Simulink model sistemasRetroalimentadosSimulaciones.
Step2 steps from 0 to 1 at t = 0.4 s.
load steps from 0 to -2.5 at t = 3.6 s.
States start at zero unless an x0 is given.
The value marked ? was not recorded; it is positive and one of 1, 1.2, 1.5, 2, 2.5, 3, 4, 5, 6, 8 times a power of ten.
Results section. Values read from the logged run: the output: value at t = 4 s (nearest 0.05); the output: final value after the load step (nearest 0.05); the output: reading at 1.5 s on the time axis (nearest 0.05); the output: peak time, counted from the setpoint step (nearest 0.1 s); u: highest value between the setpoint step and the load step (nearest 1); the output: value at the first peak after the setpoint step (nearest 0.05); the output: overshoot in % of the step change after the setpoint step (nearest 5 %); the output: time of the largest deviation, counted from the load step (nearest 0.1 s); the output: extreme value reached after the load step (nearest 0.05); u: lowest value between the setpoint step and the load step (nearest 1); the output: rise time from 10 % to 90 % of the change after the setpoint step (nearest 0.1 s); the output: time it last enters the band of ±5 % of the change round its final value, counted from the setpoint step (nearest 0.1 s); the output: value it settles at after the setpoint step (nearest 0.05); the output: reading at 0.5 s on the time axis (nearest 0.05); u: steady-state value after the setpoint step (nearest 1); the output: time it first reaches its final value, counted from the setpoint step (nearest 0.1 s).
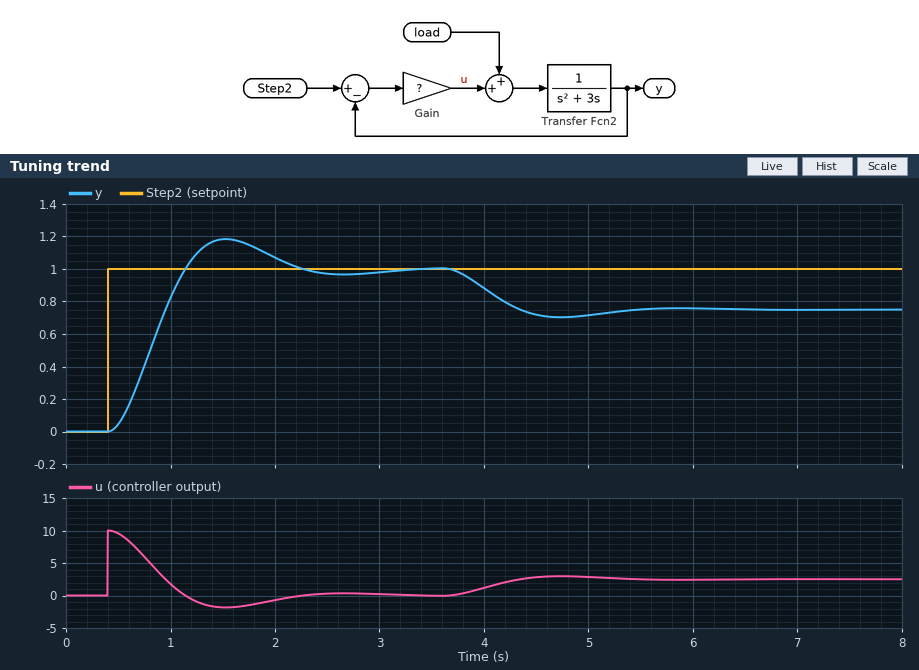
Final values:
0.90
0.75
1.20
1.1 s
10
1.20
20 %
1.1 s
0.70
-2
0.5 s
1.7 s
1.00
0.05
0
0.7 s
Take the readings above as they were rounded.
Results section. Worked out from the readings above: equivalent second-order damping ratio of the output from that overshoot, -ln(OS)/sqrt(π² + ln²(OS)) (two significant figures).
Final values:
0.46
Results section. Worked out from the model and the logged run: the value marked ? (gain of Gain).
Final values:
10
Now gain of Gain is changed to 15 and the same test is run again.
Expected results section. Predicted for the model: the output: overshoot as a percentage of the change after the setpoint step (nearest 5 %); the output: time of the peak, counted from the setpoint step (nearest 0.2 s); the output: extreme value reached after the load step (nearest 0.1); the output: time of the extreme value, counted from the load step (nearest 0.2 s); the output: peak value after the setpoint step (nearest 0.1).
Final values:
25 %
0.8 s
0.8
0.8 s
1.3
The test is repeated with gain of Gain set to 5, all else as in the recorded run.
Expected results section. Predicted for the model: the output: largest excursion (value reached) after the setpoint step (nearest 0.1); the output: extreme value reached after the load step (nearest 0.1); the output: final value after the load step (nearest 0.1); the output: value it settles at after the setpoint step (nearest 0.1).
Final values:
1.1
0.5
0.5
1.0
